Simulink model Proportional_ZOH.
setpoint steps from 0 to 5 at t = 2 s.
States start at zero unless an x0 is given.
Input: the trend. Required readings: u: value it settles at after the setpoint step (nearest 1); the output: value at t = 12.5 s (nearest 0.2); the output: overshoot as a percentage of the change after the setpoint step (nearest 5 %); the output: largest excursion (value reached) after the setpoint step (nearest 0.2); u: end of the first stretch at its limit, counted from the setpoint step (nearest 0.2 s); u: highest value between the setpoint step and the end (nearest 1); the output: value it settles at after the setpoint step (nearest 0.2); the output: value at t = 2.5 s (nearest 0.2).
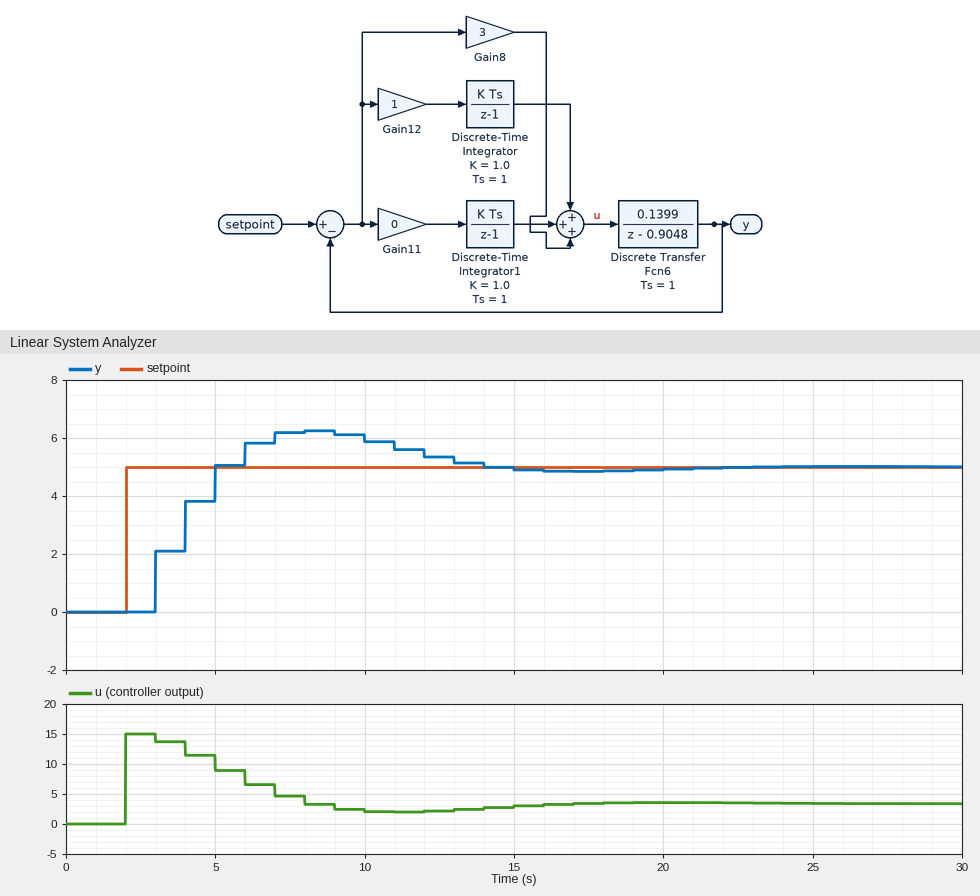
3
5.4
25 %
6.2
1.0 s
15
5.0
0.0
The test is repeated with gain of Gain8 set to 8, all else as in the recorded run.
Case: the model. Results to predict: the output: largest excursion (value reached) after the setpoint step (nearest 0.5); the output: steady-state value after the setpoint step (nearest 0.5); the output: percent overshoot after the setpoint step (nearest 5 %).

5.5
5.0
10 %
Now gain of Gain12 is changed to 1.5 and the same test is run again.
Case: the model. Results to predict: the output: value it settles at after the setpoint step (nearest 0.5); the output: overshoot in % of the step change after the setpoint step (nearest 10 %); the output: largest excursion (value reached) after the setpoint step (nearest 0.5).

5.0
40 %
7.0
